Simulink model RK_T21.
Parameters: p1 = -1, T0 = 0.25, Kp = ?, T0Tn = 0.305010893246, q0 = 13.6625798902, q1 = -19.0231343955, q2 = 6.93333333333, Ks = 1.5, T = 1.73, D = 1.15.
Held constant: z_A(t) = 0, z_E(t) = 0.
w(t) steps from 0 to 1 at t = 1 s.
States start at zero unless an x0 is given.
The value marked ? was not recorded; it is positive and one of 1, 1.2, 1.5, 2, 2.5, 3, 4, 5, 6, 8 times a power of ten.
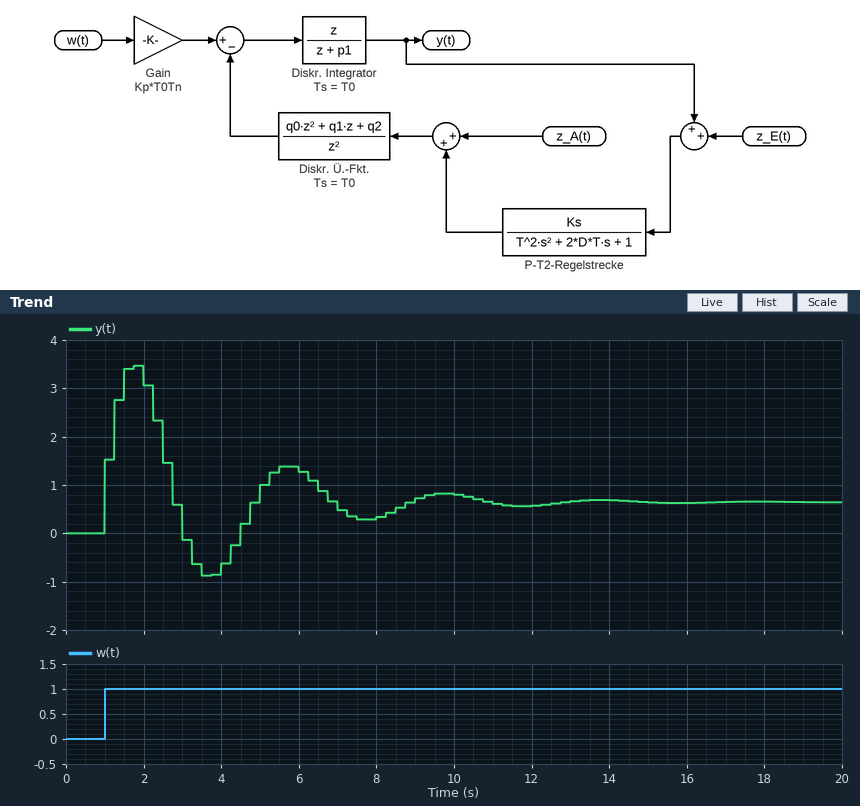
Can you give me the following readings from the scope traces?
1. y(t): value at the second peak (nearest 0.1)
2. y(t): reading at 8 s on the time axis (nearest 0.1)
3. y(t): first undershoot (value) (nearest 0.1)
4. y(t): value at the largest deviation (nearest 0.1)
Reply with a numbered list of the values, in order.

1. 1.4
2. 0.3
3. -0.9
4. 3.5
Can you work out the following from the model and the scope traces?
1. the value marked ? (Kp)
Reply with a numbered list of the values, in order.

1. 5
